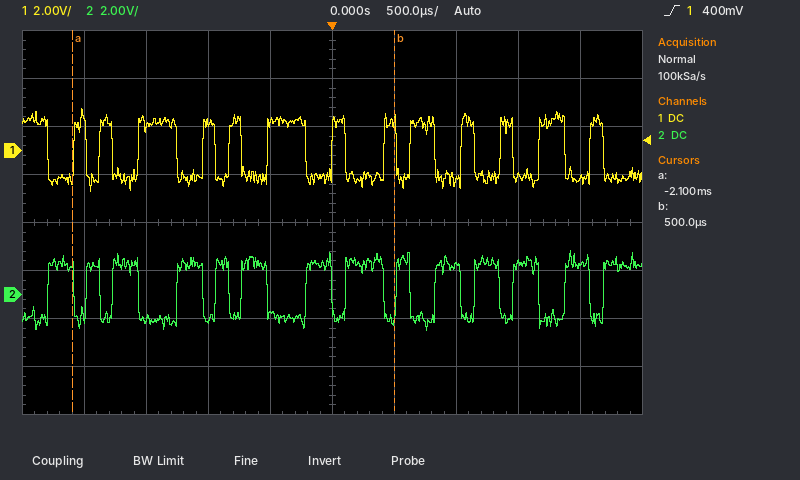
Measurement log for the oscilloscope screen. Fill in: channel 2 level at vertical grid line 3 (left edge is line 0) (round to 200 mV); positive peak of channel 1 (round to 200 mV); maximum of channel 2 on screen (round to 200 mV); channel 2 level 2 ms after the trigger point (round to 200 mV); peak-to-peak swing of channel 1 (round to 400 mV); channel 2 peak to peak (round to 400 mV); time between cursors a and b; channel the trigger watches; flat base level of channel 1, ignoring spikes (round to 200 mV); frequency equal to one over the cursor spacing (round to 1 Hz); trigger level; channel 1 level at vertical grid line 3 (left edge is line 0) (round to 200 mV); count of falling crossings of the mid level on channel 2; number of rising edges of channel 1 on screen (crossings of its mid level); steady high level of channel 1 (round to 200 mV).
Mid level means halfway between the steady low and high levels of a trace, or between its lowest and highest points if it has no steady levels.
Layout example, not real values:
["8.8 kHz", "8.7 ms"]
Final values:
["-1.0 V", "1.8 V", "1.8 V", "1.2 V", "3.6 V", "3.2 V", "2.60 ms", "channel 1", "-1.2 V", "385 Hz", "400 mV", "1.2 V", "13", "13", "1.2 V"]
